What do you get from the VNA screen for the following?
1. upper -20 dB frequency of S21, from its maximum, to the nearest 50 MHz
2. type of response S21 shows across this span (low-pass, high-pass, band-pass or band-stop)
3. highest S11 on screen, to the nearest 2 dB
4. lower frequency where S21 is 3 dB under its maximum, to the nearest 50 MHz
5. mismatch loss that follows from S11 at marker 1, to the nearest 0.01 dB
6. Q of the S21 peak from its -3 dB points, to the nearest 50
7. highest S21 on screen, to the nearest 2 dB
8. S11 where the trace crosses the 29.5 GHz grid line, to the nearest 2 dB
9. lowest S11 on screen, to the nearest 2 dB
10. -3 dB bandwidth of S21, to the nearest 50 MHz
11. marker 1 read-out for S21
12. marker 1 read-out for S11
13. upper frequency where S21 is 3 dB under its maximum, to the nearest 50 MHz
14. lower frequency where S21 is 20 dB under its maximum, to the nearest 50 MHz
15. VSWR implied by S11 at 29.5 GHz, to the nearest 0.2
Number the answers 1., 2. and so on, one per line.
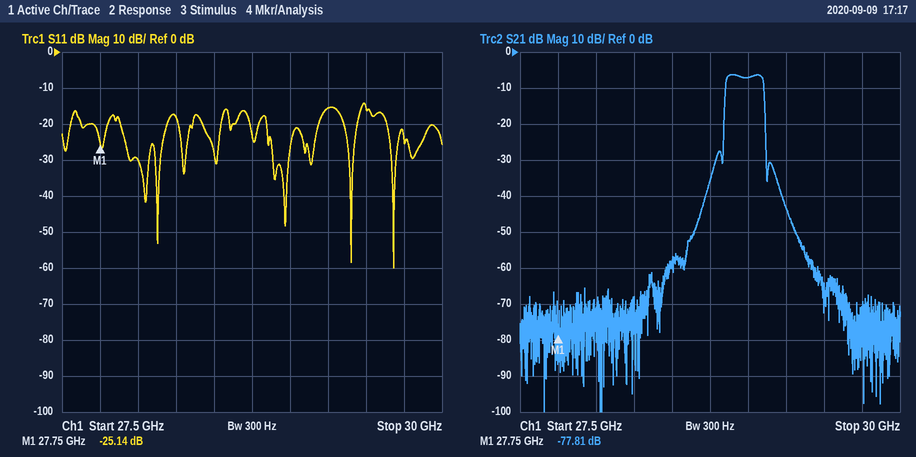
1. 29.10 GHz
2. band-pass
3. -14 dB
4. 28.85 GHz
5. 0.01 dB
6. 100
7. -6 dB
8. -16 dB
9. -60 dB
10. 250 MHz
11. -77.81 dB
12. -25.14 dB
13. 29.10 GHz
14. 28.85 GHz
15. 1.4
